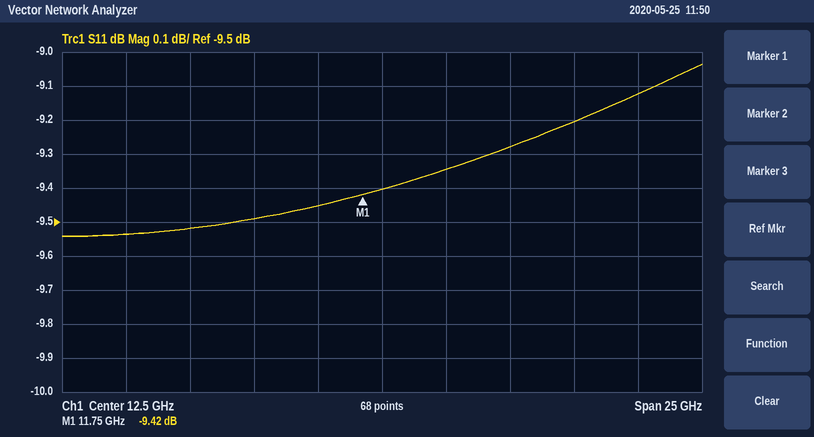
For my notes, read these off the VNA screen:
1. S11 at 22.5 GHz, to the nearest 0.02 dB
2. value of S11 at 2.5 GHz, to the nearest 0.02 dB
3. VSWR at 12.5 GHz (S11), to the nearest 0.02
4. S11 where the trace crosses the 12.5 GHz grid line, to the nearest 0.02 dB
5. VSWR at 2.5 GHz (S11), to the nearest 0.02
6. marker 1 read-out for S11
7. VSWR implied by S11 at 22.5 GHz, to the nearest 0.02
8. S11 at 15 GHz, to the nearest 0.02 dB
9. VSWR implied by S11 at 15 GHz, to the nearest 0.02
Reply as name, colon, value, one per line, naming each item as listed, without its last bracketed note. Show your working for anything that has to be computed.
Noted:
S11 at 22.5 GHz, to the nearest 0.02 dB: -9.12 dB
value of S11 at 2.5 GHz, to the nearest 0.02 dB: -9.54 dB
VSWR at 12.5 GHz (S11), to the nearest 0.02: |Γ| = 10^(-9.4/20) = 0.3388; VSWR = (1 + 0.3388)/(1 − 0.3388) ≈ 2.03, so 2.02 to the nearest 0.02
S11 where the trace crosses the 12.5 GHz grid line, to the nearest 0.02 dB: -9.40 dB
VSWR at 2.5 GHz (S11), to the nearest 0.02: |Γ| = 10^(-9.54/20) = 0.3334; VSWR = (1 + 0.3334)/(1 − 0.3334) ≈ 2.00
marker 1 read-out for S11: -9.42 dB
VSWR implied by S11 at 22.5 GHz, to the nearest 0.02: |Γ| = 10^(-9.12/20) = 0.3499; VSWR = (1 + 0.3499)/(1 − 0.3499) ≈ 2.08
S11 at 15 GHz, to the nearest 0.02 dB: -9.34 dB
VSWR implied by S11 at 15 GHz, to the nearest 0.02: |Γ| = 10^(-9.34/20) = 0.3412; VSWR = (1 + 0.3412)/(1 − 0.3412) ≈ 2.04
